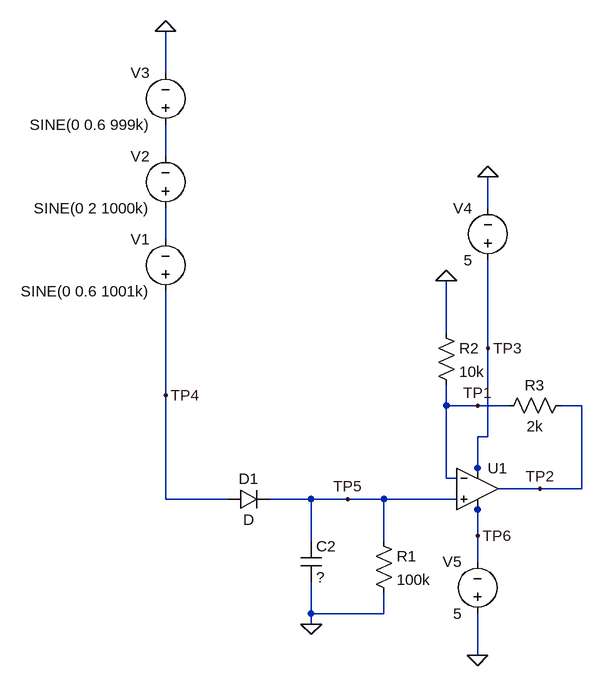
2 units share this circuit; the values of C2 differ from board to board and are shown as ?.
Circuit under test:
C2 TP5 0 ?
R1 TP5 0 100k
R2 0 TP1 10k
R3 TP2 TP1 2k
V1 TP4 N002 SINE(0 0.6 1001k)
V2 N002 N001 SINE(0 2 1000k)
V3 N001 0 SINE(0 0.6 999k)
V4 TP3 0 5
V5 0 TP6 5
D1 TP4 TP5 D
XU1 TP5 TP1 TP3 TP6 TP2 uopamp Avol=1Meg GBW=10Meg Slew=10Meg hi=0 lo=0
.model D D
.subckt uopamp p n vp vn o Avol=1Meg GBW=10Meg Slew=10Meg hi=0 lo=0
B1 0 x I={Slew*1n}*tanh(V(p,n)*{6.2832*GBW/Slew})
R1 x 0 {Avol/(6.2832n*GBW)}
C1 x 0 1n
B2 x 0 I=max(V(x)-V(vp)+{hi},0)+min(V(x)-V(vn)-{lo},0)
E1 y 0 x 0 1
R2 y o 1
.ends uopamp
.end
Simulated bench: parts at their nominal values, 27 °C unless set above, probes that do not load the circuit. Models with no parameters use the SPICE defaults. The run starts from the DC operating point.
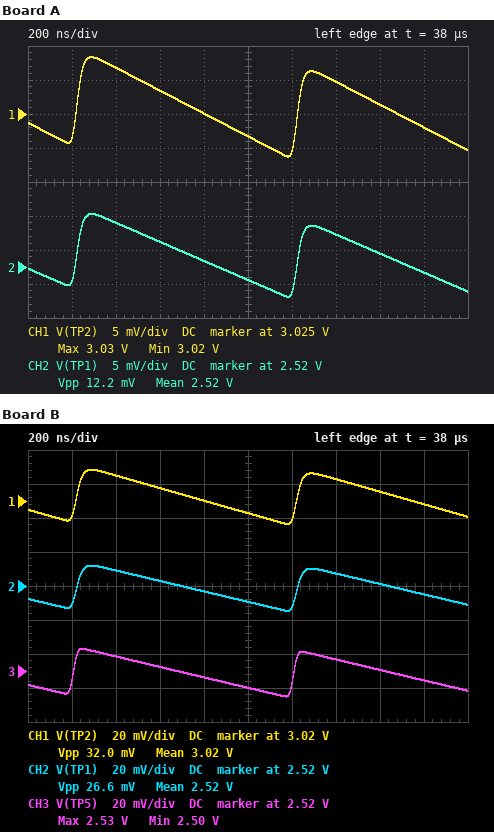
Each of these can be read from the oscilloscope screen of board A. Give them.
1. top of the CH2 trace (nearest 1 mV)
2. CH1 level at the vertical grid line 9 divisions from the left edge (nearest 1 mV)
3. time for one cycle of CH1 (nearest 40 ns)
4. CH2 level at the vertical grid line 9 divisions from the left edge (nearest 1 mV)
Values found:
2.528 V
3.023 V
1.00 µs
2.519 V
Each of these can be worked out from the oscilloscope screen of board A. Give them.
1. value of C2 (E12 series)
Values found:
1.8 nF
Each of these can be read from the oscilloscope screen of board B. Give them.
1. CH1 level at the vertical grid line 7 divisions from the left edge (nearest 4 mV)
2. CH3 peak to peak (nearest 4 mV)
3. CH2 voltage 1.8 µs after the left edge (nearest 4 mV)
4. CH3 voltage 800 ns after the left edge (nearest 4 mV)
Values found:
3.032 V
28 mV
2.516 V
2.516 V
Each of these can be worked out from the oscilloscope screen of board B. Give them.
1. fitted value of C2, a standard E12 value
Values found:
820 pF
